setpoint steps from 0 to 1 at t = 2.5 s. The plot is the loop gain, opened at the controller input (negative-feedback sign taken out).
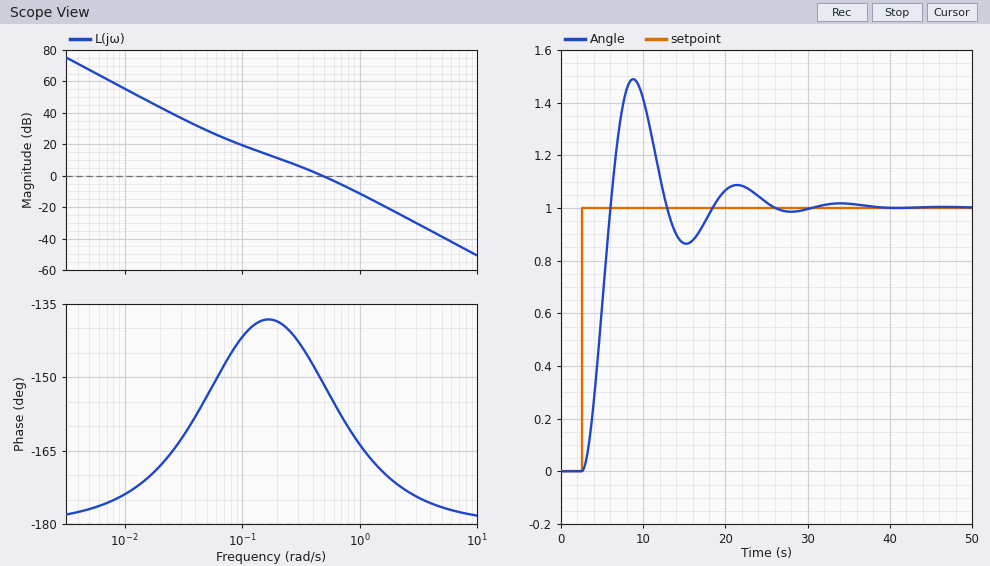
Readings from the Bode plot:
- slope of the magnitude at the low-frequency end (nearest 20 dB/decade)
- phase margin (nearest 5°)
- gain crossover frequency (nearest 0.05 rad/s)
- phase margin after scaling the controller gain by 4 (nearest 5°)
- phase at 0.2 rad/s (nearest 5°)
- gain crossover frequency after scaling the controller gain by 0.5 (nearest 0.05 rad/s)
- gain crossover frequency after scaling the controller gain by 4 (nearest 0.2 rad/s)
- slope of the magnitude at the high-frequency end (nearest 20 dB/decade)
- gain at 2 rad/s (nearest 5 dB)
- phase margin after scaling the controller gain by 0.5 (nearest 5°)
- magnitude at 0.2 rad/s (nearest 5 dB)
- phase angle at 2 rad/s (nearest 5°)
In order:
-40 dB/decade
30°
0.50 rad/s
15°
-140°
0.30 rad/s
1.0 rad/s
-40 dB/decade
-25 dB
35°
10 dB
-170°
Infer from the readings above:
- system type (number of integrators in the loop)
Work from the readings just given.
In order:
2
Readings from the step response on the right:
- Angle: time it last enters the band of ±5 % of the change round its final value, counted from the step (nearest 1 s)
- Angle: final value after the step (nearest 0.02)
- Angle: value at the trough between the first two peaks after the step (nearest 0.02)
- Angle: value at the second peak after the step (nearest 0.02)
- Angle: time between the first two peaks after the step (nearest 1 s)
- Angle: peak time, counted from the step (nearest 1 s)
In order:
21 s
1.00
0.86
1.08
13 s
6 s
